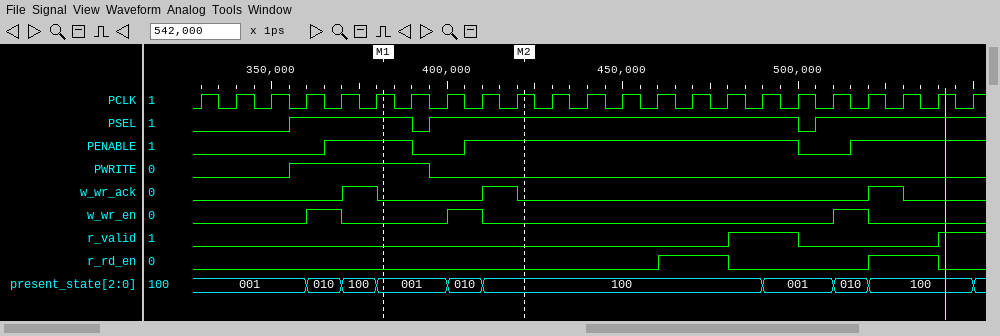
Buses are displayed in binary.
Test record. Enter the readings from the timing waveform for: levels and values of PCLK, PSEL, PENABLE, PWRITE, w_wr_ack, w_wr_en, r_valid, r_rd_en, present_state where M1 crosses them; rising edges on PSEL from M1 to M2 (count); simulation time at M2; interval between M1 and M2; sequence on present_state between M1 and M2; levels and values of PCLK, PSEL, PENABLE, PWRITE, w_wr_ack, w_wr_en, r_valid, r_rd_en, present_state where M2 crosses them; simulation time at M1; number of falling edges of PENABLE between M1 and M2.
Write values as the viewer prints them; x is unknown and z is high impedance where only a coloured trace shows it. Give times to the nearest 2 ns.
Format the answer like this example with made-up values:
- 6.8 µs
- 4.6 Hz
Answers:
- PCLK=1, PSEL=1, PENABLE=1, PWRITE=1, w_wr_ack=0, w_wr_en=0, r_valid=0, r_rd_en=0, present_state=001
- 1
- 422 ns
- 40 ns
- 001, 010, 100
- PCLK=1, PSEL=1, PENABLE=1, PWRITE=0, w_wr_ack=0, w_wr_en=0, r_valid=0, r_rd_en=0, present_state=100
- 382 ns
- 1
